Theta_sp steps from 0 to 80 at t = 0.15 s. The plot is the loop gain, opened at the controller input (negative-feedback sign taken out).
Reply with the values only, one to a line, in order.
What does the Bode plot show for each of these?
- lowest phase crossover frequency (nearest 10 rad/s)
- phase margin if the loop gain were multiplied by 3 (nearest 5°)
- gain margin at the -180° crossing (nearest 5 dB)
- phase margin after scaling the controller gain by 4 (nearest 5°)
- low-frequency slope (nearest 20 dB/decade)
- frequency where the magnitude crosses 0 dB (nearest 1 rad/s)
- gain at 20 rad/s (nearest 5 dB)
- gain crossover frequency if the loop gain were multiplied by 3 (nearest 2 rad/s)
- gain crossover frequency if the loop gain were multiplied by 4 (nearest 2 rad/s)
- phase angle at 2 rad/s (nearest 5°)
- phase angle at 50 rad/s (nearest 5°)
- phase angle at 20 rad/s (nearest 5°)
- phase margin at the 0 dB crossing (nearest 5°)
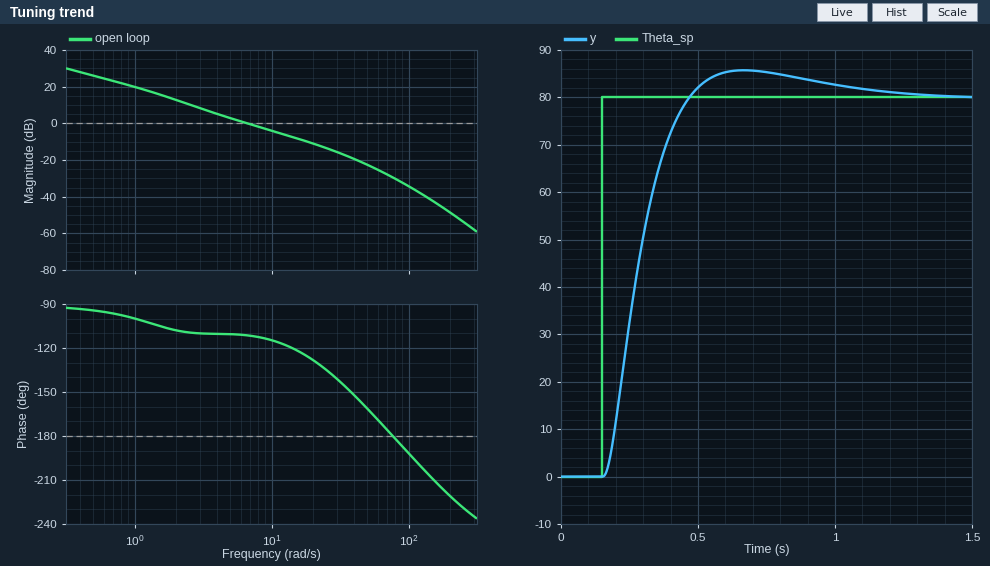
80 rad/s
55°
30 dB
50°
-20 dB/decade
7 rad/s
-10 dB
18 rad/s
22 rad/s
-110°
-160°
-130°
70°
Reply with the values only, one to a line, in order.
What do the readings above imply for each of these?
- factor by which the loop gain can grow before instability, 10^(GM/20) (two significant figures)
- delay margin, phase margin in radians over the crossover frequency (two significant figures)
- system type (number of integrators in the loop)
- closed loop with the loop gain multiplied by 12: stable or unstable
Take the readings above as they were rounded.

32
0.17 s
1
stable
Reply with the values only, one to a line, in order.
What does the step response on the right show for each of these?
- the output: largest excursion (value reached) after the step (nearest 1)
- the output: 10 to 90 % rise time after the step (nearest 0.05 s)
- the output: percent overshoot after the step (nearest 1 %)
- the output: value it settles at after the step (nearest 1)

86
0.20 s
7 %
80
